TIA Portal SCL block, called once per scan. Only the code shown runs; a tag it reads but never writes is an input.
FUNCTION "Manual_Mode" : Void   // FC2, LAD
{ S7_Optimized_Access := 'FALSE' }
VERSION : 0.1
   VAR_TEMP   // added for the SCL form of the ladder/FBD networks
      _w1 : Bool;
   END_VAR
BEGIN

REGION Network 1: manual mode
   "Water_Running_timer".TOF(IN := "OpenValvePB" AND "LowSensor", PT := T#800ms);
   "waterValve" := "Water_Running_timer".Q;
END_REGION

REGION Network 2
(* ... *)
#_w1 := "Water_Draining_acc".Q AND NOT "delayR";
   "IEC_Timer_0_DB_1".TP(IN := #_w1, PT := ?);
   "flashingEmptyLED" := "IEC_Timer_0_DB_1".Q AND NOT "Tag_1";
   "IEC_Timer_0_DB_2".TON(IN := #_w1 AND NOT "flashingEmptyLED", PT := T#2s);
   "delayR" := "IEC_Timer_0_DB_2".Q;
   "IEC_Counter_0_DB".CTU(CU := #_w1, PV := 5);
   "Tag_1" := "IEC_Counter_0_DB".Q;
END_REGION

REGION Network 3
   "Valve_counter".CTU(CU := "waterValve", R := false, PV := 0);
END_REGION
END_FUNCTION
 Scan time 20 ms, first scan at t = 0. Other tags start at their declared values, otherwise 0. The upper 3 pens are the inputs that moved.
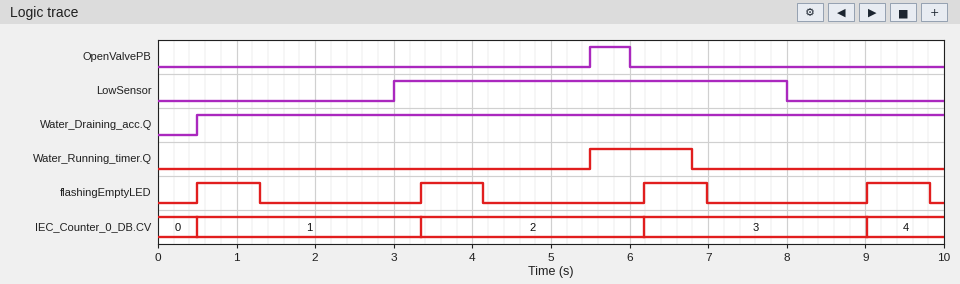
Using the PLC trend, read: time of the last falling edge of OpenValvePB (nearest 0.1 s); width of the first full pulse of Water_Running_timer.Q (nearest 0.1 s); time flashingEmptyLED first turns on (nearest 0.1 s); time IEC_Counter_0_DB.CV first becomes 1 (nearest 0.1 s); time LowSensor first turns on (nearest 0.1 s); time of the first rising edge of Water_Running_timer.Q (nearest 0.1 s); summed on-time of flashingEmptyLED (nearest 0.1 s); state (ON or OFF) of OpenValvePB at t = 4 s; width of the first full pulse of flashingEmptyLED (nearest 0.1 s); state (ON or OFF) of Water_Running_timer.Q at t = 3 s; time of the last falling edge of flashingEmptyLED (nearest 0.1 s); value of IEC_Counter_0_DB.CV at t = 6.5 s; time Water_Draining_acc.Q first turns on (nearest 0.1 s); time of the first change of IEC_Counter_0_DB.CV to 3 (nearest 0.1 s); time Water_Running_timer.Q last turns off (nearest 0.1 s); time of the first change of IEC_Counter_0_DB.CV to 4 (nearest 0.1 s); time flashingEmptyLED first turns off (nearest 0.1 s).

6.0 s
1.3 s
0.5 s
0.5 s
3.0 s
5.5 s
3.2 s
OFF
0.8 s
OFF
9.8 s
3
0.5 s
6.2 s
6.8 s
9.0 s
1.3 s
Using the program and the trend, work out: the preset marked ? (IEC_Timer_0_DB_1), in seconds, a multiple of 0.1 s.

0.8 s
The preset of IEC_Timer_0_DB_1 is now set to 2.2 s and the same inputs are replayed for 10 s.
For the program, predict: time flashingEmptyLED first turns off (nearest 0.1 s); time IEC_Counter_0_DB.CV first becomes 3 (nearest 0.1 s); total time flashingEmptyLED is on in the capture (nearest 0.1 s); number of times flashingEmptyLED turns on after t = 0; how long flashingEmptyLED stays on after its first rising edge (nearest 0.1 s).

2.7 s
9.0 s
5.4 s
3
2.2 s
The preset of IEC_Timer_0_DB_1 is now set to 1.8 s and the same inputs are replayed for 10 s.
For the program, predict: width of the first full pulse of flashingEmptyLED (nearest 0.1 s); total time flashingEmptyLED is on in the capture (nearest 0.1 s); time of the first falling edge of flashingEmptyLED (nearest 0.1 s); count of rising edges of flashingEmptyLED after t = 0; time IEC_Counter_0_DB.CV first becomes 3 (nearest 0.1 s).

1.8 s
5.4 s
2.3 s
3
8.2 s
